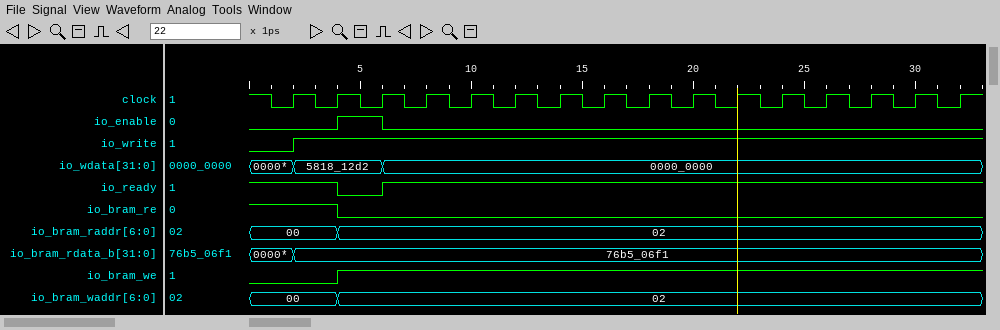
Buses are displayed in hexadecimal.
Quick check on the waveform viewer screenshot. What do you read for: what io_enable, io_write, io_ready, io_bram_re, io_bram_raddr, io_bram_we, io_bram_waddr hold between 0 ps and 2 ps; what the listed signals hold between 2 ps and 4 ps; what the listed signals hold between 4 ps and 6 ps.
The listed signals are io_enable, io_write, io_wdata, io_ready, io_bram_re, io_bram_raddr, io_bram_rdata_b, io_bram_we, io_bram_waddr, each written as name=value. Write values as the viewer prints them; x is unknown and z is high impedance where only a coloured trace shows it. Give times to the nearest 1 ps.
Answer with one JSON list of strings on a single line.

["io_enable=0, io_write=0, io_ready=1, io_bram_re=1, io_bram_raddr=00, io_bram_we=0, io_bram_waddr=00", "io_enable=0, io_write=1, io_wdata=5818_12d2, io_ready=1, io_bram_re=1, io_bram_raddr=00, io_bram_rdata_b=76b5_06f1, io_bram_we=0, io_bram_waddr=00", "io_enable=1, io_write=1, io_wdata=5818_12d2, io_ready=0, io_bram_re=0, io_bram_raddr=02, io_bram_rdata_b=76b5_06f1, io_bram_we=1, io_bram_waddr=02"]
